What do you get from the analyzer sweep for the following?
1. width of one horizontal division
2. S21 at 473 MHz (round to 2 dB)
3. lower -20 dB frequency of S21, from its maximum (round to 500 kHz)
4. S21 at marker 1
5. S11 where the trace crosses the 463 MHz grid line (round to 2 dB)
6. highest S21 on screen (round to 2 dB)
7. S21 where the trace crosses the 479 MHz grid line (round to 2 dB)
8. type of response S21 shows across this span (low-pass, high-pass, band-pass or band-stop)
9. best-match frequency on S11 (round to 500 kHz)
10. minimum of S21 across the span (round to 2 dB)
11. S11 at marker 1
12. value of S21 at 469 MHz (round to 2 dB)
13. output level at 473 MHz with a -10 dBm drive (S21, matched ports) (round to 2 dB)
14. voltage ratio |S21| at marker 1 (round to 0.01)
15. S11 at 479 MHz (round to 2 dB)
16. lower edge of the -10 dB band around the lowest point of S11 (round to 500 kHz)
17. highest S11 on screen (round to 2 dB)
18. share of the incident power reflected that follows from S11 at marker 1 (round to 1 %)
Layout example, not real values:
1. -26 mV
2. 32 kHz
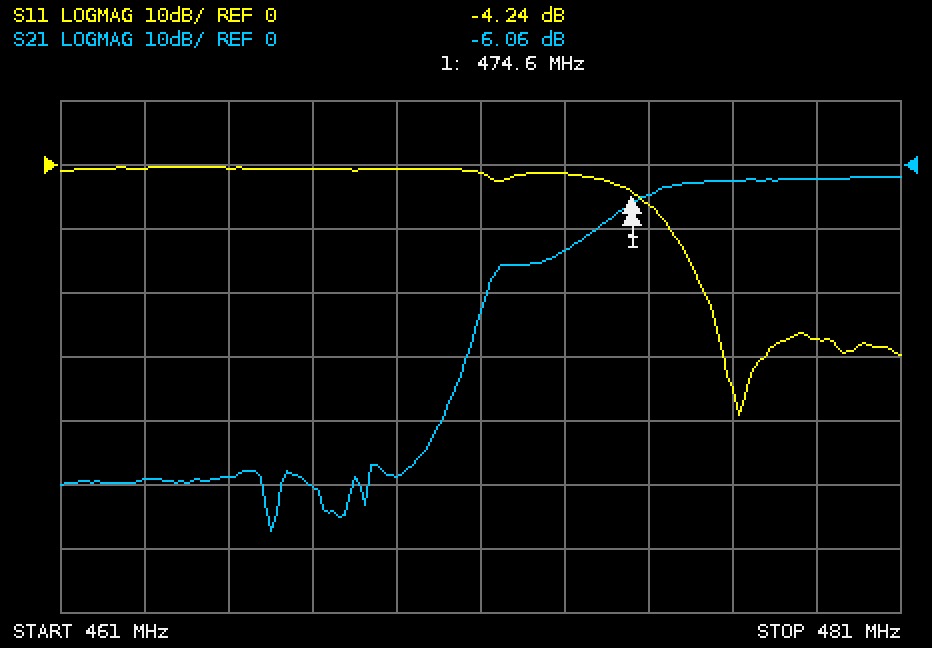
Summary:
1. 2 MHz
2. -14 dB
3. 471.0 MHz
4. -6.06 dB
5. 0 dB
6. -2 dB
7. -2 dB
8. high-pass
9. 477.0 MHz
10. -58 dB
11. -4.24 dB
12. -48 dB
13. -24 dBm
14. 0.50
15. -28 dB
16. 475.5 MHz
17. 0 dB
18. 38 %
